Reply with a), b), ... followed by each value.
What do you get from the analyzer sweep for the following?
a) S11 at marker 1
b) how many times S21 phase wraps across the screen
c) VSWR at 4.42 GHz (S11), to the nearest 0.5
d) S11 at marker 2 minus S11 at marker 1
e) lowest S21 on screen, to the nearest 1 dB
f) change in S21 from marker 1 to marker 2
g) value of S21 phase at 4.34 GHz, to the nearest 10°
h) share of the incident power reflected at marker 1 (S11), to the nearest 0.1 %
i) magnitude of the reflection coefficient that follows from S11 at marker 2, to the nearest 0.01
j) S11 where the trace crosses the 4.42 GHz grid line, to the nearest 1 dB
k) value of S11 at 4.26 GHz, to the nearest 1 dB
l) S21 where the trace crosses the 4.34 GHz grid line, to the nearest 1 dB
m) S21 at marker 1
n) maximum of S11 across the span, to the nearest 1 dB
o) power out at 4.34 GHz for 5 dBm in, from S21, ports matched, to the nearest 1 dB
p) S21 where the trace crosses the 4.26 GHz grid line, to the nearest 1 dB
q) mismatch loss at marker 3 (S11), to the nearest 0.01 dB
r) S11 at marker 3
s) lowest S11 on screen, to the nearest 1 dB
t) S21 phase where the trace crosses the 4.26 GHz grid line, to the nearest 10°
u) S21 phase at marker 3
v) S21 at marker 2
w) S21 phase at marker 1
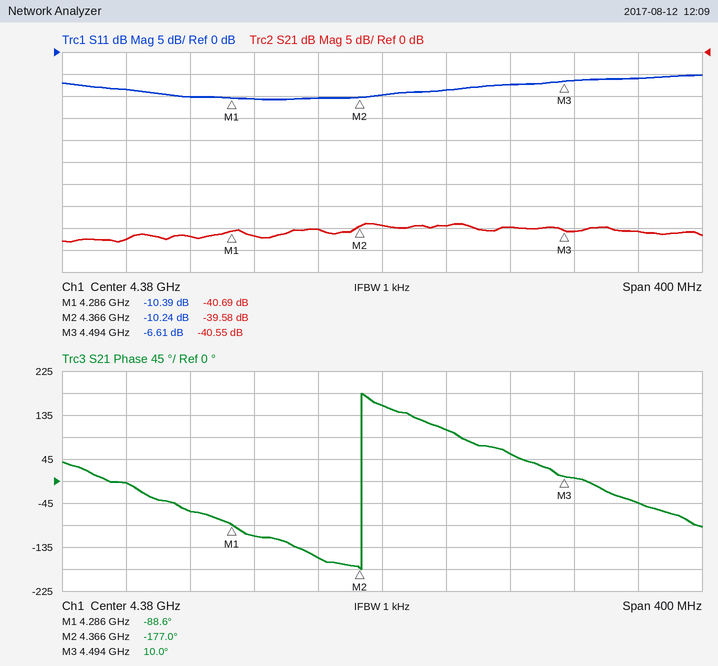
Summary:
a) -10.39 dB
b) 1
c) 2.0
d) 0.15 dB
e) -43 dB
f) 1.11 dB
g) -160°
h) 9.1 %
i) 0.31
j) -9 dB
k) -10 dB
l) -40 dB
m) -40.69 dB
n) -5 dB
o) -35 dBm
p) -42 dB
q) 1.07 dB
r) -6.61 dB
s) -11 dB
t) -60°
u) 10.0°
v) -39.58 dB
w) -88.6°
